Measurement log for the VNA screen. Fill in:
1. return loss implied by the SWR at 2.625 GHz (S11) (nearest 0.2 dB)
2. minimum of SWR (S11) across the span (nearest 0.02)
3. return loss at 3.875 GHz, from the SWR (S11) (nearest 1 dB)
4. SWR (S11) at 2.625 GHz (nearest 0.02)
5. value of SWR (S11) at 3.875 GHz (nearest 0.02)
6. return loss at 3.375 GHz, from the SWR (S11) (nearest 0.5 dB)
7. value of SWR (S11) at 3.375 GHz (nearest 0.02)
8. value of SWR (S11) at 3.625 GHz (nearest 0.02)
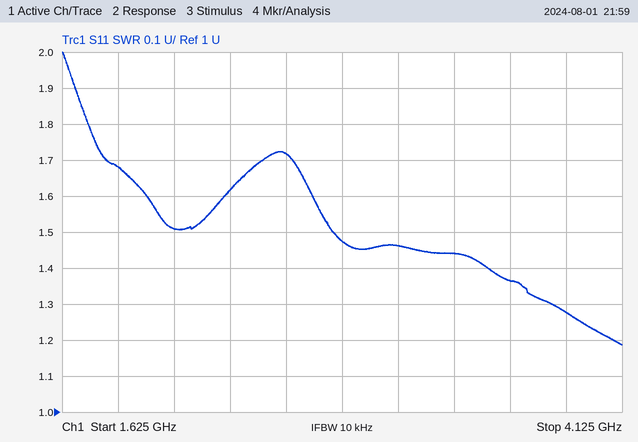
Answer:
11.6 dB
1.18
18 dB
1.72
1.28
15.0 dB
1.44
1.36
